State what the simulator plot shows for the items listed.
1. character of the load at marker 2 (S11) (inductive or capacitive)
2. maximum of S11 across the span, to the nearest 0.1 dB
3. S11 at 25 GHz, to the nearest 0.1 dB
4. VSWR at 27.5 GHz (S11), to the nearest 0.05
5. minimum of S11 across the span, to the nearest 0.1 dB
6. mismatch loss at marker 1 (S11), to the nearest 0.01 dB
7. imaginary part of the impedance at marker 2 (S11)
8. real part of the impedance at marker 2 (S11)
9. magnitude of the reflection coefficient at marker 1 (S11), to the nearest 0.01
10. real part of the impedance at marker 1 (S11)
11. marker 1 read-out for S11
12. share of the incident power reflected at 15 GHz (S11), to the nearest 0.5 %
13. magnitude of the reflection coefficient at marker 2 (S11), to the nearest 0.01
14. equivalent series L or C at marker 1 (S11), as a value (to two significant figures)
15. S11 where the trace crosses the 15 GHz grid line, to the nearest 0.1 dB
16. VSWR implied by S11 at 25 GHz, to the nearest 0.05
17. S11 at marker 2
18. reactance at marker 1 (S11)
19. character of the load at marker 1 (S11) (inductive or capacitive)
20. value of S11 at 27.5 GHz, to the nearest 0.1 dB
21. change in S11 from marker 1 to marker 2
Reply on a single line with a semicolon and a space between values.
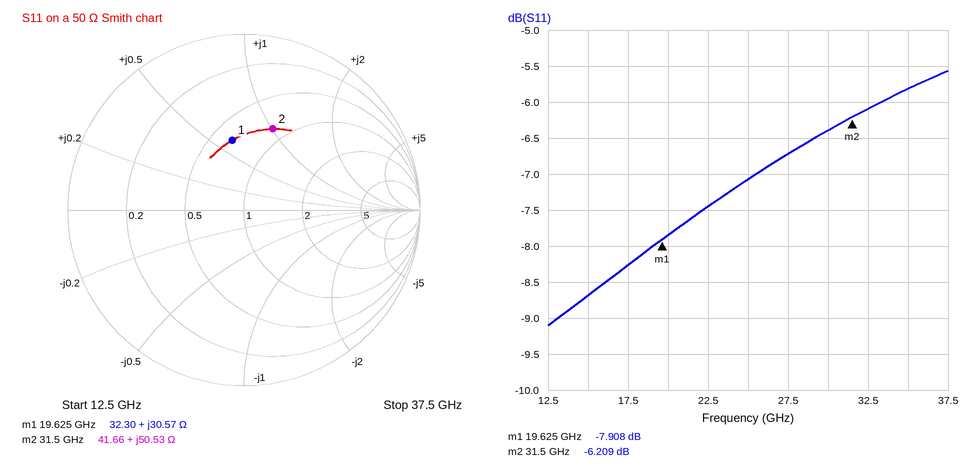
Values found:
inductive; -5.6 dB; -7.1 dB; 2.70; -9.1 dB; 0.77 dB; +50.53 Ω; 41.66 Ω; 0.40; 32.30 Ω; -7.908 dB; 13.5 %; 0.49; 250 pH; -8.7 dB; 2.60; -6.209 dB; +30.57 Ω; inductive; -6.7 dB; 1.699 dB
